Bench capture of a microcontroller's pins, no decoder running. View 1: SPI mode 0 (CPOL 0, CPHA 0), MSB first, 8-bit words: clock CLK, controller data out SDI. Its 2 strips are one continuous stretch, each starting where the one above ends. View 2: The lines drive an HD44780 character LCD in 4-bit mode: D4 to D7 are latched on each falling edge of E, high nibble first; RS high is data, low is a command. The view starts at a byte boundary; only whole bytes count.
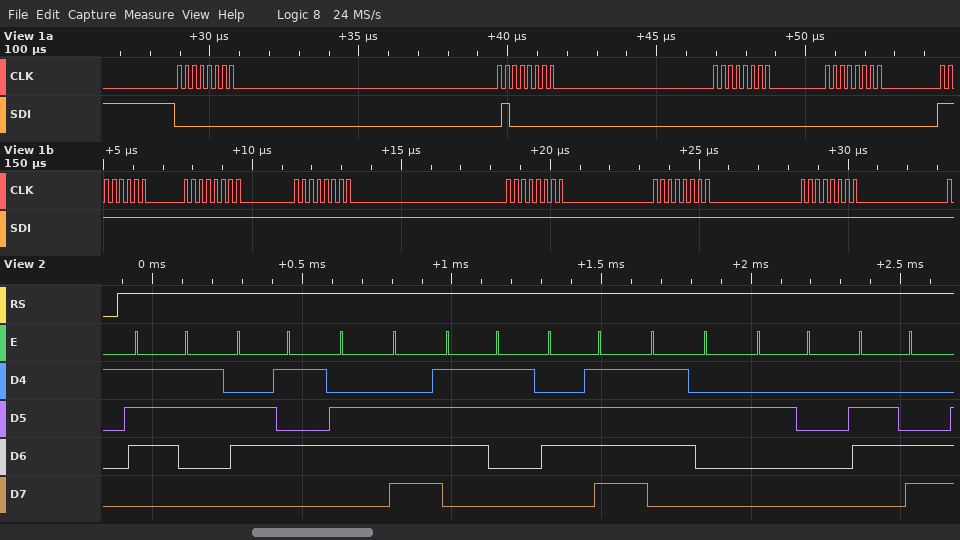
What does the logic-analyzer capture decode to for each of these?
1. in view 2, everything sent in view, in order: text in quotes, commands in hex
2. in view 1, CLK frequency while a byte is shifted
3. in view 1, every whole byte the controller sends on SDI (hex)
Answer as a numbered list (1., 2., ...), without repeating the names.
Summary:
1. "sensor l"
2. 4 MHz
3. 0x00 0x40 0x00 0x00 0xFF 0xFF 0xFF 0xFF 0xFF 0xFF
